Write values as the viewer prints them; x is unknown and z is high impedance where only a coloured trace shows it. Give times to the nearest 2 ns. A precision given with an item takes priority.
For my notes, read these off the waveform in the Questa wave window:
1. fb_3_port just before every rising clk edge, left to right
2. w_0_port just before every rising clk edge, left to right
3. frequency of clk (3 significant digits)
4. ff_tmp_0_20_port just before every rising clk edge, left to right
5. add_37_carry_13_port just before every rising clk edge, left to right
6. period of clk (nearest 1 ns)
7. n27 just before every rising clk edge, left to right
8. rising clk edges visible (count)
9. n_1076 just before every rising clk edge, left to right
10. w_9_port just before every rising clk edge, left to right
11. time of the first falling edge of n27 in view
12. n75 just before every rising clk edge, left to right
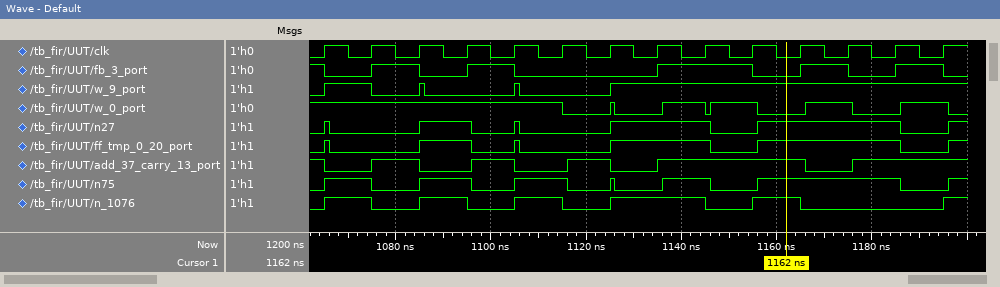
1 0 1 0 1 0 0 0 1 1 0 1 0 1
1 1 1 1 1 1 0 0 1 1 0 1 0 1
100 MHz
0 0 0 1 0 0 0 1 1 0 1 1 1 0
1 0 1 0 1 0 1 0 1 1 1 0 1 1
10 ns
0 0 0 1 0 0 0 1 1 0 1 1 1 0
14
0 1 0 1 0 1 0 1 1 0 1 0 0 0
0 1 0 0 0 0 0 1 1 1 1 1 1 1
1066 ns
0 1 0 1 0 1 0 0 1 0 1 1 1 0
